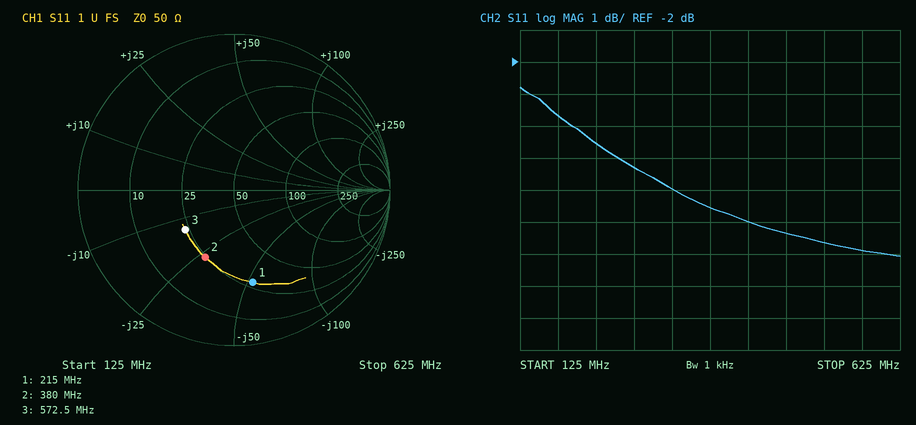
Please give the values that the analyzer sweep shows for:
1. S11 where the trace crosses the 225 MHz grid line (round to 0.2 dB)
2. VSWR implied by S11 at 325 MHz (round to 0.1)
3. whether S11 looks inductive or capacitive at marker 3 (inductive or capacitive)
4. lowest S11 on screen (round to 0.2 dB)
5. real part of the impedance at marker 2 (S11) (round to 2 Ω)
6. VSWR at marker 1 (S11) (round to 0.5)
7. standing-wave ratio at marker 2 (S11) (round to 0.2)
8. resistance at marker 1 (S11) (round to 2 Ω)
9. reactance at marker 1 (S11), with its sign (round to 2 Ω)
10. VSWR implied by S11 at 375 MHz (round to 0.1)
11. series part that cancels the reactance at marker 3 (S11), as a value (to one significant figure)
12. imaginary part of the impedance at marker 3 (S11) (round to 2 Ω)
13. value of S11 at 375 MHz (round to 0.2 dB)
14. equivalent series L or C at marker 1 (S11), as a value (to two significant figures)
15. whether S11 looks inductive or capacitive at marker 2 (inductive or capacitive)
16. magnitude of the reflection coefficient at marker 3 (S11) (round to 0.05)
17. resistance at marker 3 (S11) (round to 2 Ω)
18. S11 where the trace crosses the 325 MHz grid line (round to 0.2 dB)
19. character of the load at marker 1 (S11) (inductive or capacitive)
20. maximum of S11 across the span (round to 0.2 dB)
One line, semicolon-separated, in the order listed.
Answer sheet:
-4.6 dB; 3.0; capacitive; -8.0 dB; 24 Ω; 4.0; 2.8; 28 Ω; -52 Ω; 2.8; 4 nH; -14 Ω; -6.6 dB; 14 pF; capacitive; 0.40; 24 Ω; -6.0 dB; capacitive; -2.8 dB
